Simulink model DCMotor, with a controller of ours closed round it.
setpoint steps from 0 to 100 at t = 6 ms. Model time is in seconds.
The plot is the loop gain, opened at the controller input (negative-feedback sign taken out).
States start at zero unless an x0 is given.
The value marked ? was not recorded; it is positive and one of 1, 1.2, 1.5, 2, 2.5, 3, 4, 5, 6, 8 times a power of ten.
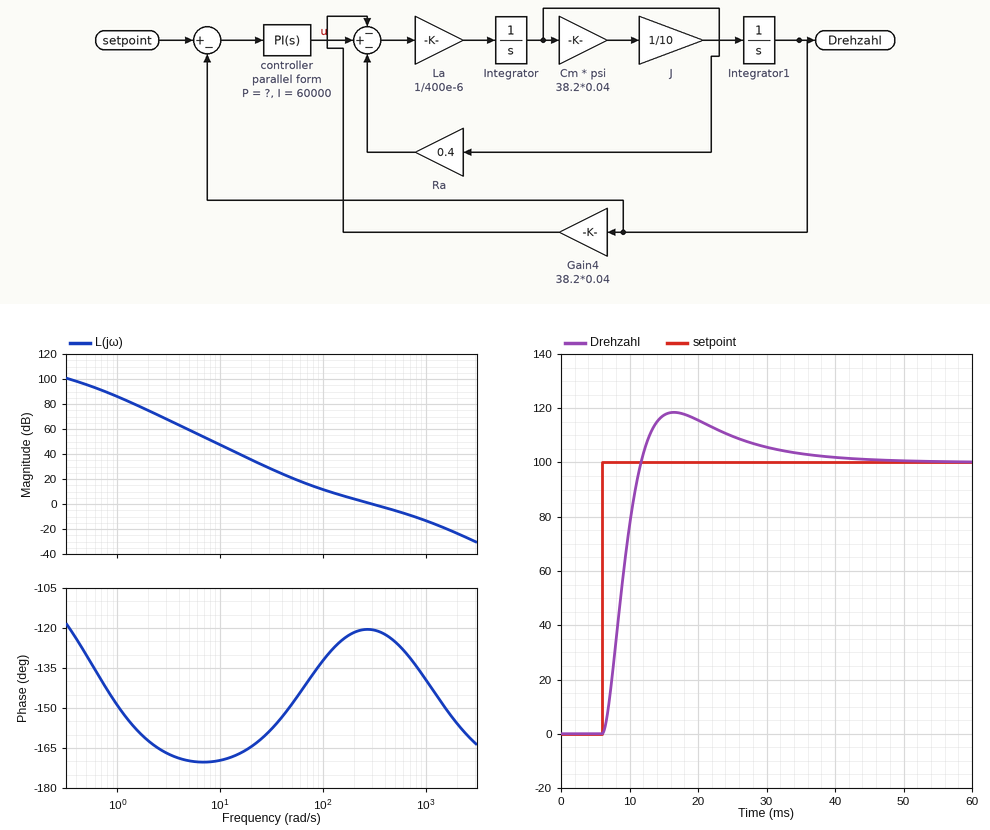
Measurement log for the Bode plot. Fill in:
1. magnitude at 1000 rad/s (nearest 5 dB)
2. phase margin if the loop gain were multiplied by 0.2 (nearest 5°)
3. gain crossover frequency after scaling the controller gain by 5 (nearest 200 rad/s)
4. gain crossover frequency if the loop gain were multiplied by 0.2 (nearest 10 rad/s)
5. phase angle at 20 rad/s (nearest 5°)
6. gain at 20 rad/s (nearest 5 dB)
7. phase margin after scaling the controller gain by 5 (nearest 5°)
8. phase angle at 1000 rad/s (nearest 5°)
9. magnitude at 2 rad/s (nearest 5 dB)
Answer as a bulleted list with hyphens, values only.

- -15 dB
- 45°
- 1000 rad/s
- 80 rad/s
- -165°
- 35 dB
- 40°
- -140°
- 75 dB
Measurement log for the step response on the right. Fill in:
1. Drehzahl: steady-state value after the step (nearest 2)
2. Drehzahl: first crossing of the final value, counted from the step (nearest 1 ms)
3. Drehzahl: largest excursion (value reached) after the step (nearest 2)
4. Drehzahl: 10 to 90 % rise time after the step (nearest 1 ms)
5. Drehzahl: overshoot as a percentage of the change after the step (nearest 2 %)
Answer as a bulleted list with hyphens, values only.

- 100
- 6 ms
- 118
- 4 ms
- 18 %
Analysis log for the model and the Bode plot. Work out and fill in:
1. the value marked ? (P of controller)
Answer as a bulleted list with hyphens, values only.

- 800
